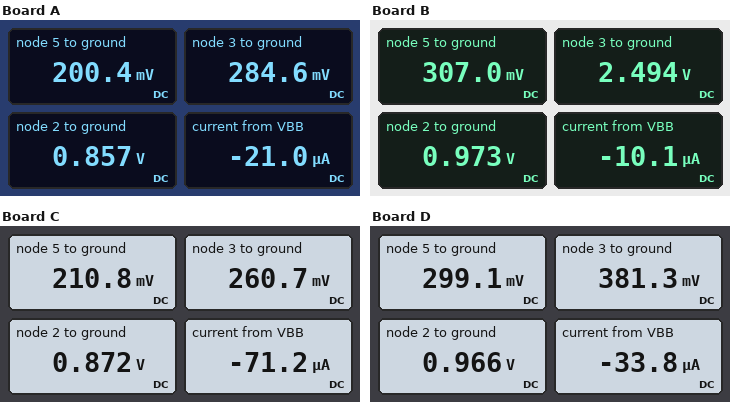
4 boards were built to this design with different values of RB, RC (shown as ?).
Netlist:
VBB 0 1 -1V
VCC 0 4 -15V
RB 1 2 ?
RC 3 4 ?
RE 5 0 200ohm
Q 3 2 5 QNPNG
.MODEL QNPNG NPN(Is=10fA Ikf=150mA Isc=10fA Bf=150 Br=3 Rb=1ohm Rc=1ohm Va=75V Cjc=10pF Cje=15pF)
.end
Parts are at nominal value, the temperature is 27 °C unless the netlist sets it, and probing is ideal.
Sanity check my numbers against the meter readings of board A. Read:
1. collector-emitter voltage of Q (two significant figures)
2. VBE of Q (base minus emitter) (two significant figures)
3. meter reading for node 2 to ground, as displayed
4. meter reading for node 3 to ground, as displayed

84 mV
660 mV
0.857 V
284.6 mV
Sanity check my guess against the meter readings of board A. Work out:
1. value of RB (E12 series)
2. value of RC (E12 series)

6.8 kΩ
15 kΩ
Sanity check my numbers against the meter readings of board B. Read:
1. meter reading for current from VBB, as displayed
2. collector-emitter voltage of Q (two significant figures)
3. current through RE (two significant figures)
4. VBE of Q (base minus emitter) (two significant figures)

-10.1 µA
2.2 V
1.5 mA
670 mV
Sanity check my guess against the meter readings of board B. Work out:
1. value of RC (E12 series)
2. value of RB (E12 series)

8.2 kΩ
2.7 kΩ
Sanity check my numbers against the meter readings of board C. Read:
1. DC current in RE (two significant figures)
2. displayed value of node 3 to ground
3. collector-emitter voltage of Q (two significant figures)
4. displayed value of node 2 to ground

1.1 mA
260.7 mV
50 mV
0.872 V
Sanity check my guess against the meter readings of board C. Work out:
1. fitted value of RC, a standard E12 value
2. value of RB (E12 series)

15 kΩ
1.8 kΩ
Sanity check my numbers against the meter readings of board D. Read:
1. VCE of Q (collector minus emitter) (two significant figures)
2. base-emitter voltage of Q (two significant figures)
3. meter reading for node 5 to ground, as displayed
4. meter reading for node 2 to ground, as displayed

82 mV
670 mV
299.1 mV
0.966 V
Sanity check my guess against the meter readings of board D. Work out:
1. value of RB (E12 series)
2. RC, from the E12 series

1 kΩ
10 kΩ
